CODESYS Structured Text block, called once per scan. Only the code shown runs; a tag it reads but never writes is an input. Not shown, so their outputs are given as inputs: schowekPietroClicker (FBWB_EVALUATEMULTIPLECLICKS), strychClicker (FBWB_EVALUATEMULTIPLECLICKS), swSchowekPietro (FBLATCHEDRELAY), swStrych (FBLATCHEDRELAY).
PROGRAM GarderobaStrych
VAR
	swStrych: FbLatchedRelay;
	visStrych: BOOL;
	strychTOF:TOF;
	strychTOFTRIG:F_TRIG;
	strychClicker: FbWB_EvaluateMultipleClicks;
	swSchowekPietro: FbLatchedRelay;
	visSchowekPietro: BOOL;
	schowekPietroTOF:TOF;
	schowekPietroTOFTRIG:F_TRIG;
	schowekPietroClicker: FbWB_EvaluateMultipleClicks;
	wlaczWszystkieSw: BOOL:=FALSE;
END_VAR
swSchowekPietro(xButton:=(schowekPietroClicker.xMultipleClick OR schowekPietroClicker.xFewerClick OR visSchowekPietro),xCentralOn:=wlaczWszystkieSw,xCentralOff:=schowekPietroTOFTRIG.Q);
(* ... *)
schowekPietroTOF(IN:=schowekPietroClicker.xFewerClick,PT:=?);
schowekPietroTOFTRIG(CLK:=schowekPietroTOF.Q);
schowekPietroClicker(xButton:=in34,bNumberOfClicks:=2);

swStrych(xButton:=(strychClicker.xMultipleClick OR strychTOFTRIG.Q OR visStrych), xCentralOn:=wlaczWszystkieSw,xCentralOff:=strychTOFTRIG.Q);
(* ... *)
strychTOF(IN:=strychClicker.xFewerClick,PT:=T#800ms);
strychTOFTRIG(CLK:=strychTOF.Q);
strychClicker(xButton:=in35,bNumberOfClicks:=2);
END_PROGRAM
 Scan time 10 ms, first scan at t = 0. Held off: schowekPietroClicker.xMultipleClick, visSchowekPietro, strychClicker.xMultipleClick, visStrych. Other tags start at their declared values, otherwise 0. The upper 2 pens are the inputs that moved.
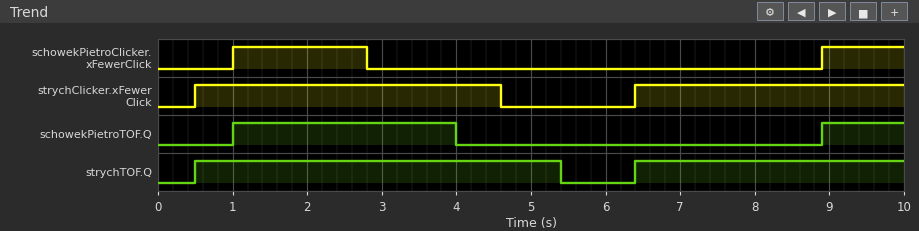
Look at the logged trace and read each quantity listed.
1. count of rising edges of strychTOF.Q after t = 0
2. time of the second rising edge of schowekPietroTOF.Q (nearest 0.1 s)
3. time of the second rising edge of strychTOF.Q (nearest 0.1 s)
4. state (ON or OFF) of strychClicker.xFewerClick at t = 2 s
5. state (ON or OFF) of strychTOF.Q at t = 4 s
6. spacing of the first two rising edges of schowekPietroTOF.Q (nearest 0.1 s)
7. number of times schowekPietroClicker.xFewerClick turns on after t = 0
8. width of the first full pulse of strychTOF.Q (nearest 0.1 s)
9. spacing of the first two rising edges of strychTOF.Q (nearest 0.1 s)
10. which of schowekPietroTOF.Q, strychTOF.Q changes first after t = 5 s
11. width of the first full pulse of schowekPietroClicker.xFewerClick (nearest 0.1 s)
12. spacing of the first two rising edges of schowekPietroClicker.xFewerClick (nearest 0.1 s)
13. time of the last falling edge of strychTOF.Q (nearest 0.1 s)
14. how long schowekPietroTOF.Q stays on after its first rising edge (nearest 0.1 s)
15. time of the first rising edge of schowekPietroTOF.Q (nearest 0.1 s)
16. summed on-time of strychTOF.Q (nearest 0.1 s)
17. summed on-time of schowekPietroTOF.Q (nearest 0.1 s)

2
8.9 s
6.4 s
ON
ON
7.9 s
2
4.9 s
5.9 s
strychTOF.Q
1.8 s
7.9 s
5.4 s
3.0 s
1.0 s
8.5 s
4.1 s
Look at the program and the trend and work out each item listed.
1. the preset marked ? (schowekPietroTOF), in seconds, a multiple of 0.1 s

1.2 s
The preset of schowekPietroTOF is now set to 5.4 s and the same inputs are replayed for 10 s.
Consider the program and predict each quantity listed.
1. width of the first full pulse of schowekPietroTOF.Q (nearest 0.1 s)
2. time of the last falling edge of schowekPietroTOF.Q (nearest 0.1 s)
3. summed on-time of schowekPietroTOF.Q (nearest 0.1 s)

7.2 s
8.2 s
8.3 s
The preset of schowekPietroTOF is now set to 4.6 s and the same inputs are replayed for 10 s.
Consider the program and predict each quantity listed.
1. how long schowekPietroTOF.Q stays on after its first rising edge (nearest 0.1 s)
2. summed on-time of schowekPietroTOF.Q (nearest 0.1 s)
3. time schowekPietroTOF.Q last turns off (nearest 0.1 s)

6.4 s
7.5 s
7.4 s
